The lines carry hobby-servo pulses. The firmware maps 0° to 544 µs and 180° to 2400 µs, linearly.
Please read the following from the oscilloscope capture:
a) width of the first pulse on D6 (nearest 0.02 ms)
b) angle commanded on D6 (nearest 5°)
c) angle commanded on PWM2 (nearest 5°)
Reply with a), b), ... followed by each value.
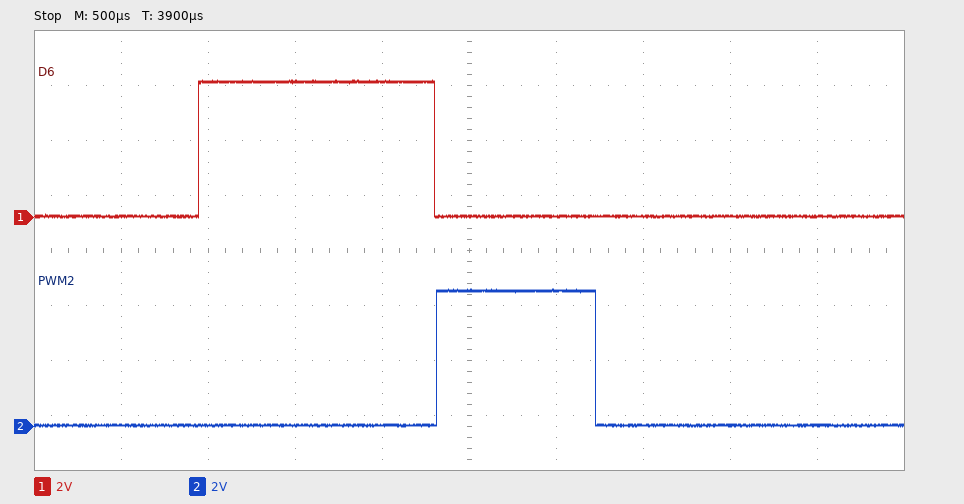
a) 1.36 ms
b) 80°
c) 35°
